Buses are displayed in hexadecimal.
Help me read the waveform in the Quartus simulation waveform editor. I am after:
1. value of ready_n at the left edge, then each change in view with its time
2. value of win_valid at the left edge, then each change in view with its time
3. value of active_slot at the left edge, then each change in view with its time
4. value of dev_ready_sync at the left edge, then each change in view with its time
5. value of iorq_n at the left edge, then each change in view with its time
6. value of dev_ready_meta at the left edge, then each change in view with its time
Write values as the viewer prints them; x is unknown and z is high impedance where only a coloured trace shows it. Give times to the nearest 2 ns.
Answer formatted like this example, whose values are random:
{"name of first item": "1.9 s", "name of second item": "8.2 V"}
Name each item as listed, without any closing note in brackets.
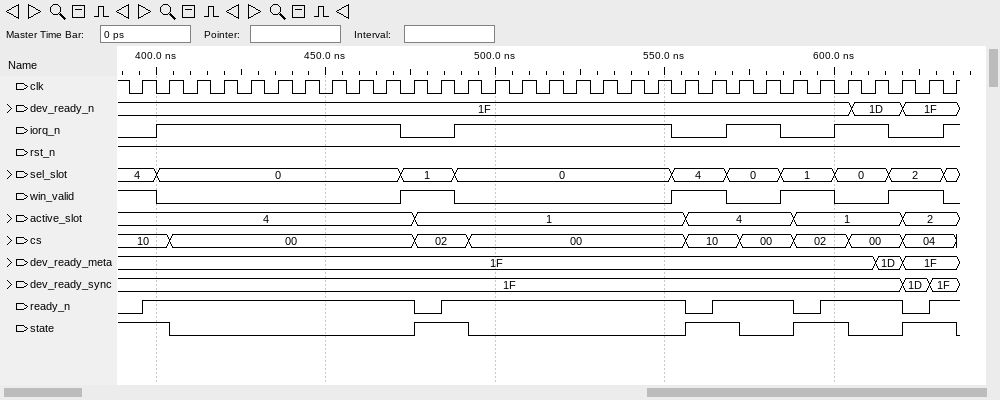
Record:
{"value of ready_n at the left edge, then each change in view with its time": "0, 1 at 396 ns, 0 at 476 ns, 1 at 484 ns, 0 at 556 ns, 1 at 564 ns, 0 at 588 ns, 1 at 596 ns, 0 at 620 ns, 1 at 628 ns", "value of win_valid at the left edge, then each change in view with its time": "1, 0 at 400 ns, 1 at 472 ns, 0 at 488 ns, 1 at 552 ns, 0 at 568 ns, 1 at 584 ns, 0 at 600 ns, 1 at 616 ns, 0 at 632 ns", "value of active_slot at the left edge, then each change in view with its time": "4, 1 at 476 ns, 4 at 556 ns, 1 at 588 ns, 2 at 620 ns", "value of dev_ready_sync at the left edge, then each change in view with its time": "1F, 1D at 620 ns, 1F at 628 ns", "value of iorq_n at the left edge, then each change in view with its time": "0, 1 at 400 ns, 0 at 472 ns, 1 at 488 ns, 0 at 552 ns, 1 at 568 ns, 0 at 584 ns, 1 at 600 ns, 0 at 616 ns, 1 at 632 ns", "value of dev_ready_meta at the left edge, then each change in view with its time": "1F, 1D at 612 ns, 1F at 620 ns"}
